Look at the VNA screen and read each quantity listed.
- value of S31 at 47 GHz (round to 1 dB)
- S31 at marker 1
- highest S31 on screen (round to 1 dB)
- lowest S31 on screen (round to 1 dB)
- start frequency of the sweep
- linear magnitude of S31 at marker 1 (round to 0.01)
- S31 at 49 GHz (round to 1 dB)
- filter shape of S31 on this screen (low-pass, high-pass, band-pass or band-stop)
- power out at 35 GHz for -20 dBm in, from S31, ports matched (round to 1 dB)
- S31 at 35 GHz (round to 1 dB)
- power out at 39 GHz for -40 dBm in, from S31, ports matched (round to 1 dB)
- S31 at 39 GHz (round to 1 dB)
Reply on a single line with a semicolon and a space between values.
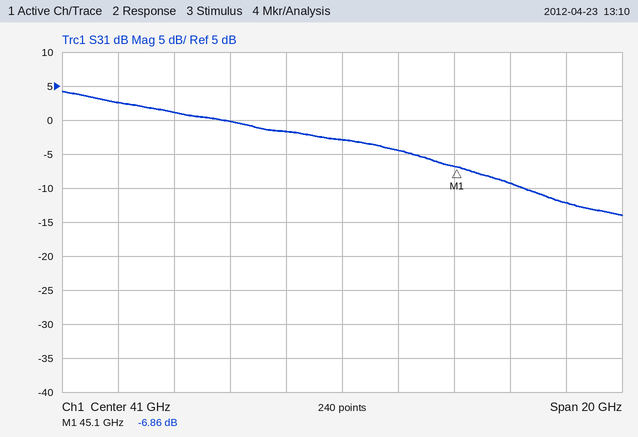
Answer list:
-9 dB; -6.86 dB; 4 dB; -14 dB; 31 GHz; 0.45; -12 dB; low-pass; -19 dBm; 1 dB; -42 dBm; -2 dB
